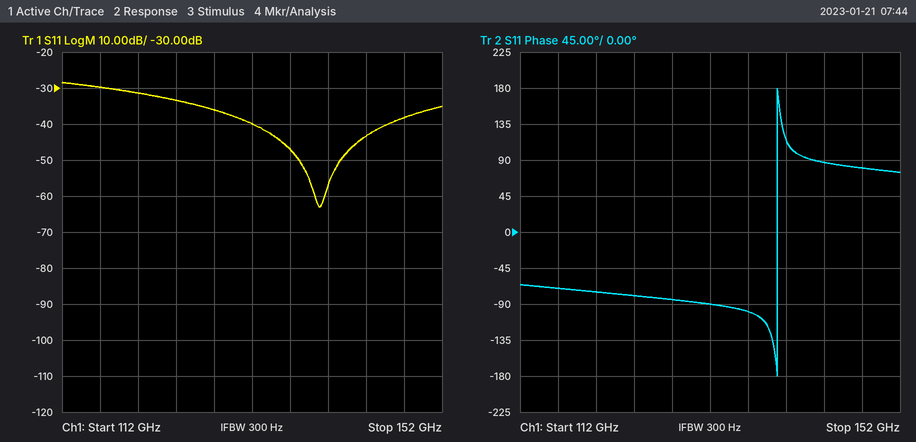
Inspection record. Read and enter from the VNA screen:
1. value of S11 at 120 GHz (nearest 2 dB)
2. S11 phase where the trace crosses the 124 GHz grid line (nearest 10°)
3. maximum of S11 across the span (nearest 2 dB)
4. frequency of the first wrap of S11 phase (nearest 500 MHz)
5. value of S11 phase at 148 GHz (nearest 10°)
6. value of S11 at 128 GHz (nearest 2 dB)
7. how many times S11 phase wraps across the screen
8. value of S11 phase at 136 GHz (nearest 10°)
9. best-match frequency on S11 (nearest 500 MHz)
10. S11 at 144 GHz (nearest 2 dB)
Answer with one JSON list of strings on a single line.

["-32 dB", "-80°", "-28 dB", "139.0 GHz", "80°", "-36 dB", "1", "-100°", "139.0 GHz", "-44 dB"]
